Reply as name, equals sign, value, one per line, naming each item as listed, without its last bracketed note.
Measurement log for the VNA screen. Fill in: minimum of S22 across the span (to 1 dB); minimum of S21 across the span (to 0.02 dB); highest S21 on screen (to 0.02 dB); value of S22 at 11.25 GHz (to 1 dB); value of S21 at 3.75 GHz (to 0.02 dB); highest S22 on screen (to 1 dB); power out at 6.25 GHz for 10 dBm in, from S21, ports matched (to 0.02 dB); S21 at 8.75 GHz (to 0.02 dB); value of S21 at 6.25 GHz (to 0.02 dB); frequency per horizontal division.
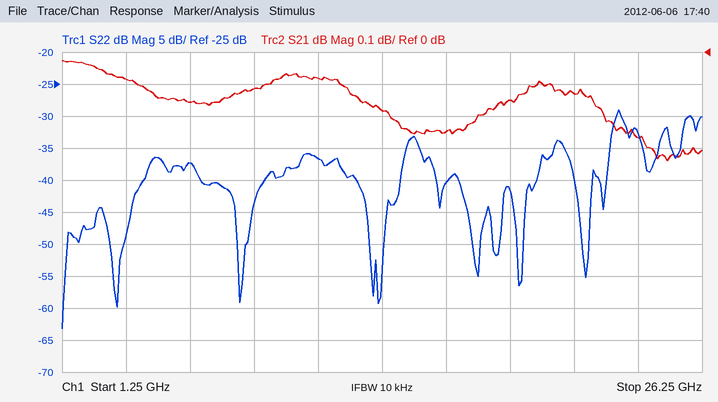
minimum of S22 across the span = -63 dB
minimum of S21 across the span = -0.34 dB
highest S21 on screen = -0.02 dB
value of S22 at 11.25 GHz = -37 dB
value of S21 at 3.75 GHz = -0.08 dB
highest S22 on screen = -29 dB
power out at 6.25 GHz for 10 dBm in, from S21, ports matched = 9.84 dBm
S21 at 8.75 GHz = -0.12 dB
value of S21 at 6.25 GHz = -0.16 dB
frequency per horizontal division = 2.5 GHz
